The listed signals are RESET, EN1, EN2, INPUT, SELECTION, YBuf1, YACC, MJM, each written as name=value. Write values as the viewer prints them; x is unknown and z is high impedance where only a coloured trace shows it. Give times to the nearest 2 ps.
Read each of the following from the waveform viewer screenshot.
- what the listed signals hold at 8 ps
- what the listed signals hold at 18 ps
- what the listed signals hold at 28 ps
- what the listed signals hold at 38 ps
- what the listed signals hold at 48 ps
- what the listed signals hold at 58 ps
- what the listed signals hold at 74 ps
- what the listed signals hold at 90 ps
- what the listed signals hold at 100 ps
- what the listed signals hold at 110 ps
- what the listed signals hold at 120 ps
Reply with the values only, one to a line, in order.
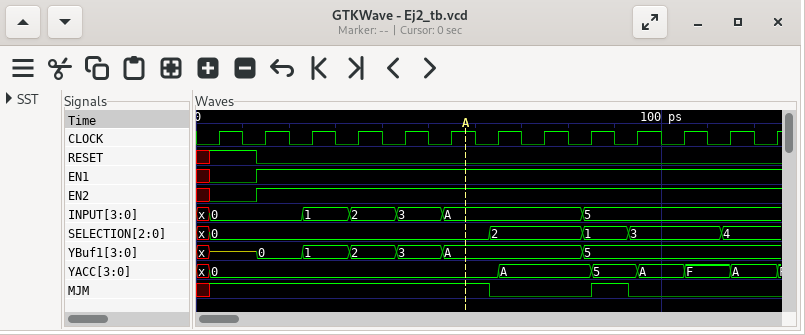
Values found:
RESET=1, EN1=0, EN2=0, INPUT=0, SELECTION=0, YBuf1=z, YACC=0, MJM=1
RESET=0, EN1=1, EN2=1, INPUT=0, SELECTION=0, YBuf1=0, YACC=0, MJM=1
RESET=0, EN1=1, EN2=1, INPUT=1, SELECTION=0, YBuf1=1, YACC=0, MJM=1
RESET=0, EN1=1, EN2=1, INPUT=2, SELECTION=0, YBuf1=2, YACC=0, MJM=1
RESET=0, EN1=1, EN2=1, INPUT=3, SELECTION=0, YBuf1=3, YACC=0, MJM=1
RESET=0, EN1=1, EN2=1, INPUT=A, SELECTION=0, YBuf1=A, YACC=0, MJM=1
RESET=0, EN1=1, EN2=1, INPUT=A, SELECTION=2, YBuf1=A, YACC=A, MJM=0
RESET=0, EN1=1, EN2=1, INPUT=5, SELECTION=1, YBuf1=5, YACC=5, MJM=1
RESET=0, EN1=1, EN2=1, INPUT=5, SELECTION=3, YBuf1=5, YACC=A, MJM=0
RESET=0, EN1=1, EN2=1, INPUT=5, SELECTION=3, YBuf1=5, YACC=F, MJM=0
RESET=0, EN1=1, EN2=1, INPUT=5, SELECTION=4, YBuf1=5, YACC=A, MJM=0
